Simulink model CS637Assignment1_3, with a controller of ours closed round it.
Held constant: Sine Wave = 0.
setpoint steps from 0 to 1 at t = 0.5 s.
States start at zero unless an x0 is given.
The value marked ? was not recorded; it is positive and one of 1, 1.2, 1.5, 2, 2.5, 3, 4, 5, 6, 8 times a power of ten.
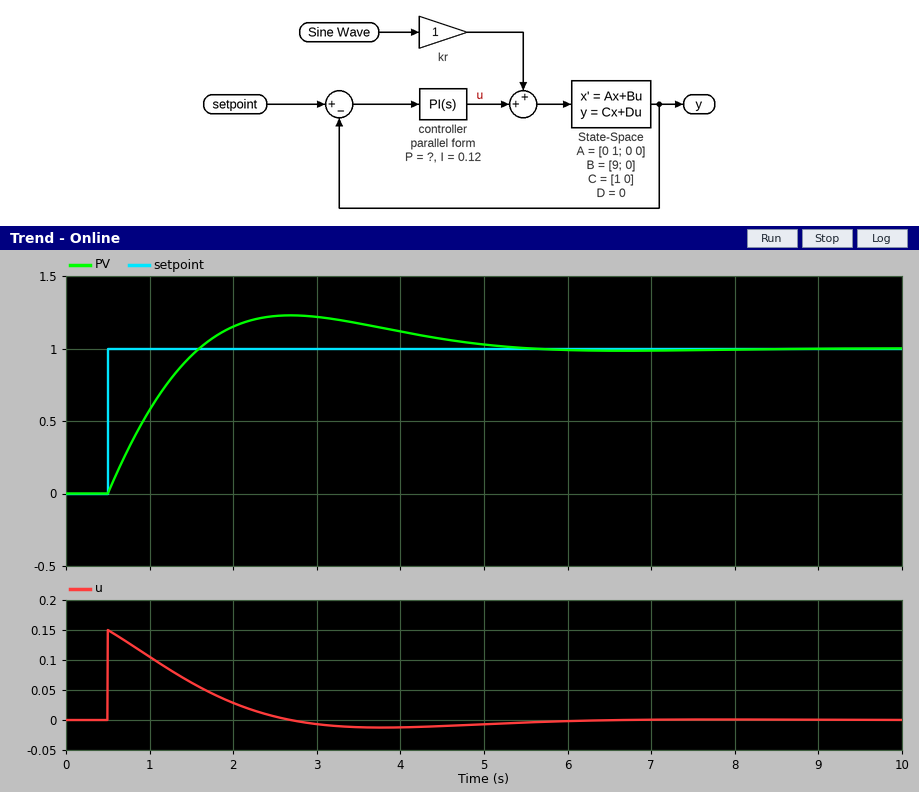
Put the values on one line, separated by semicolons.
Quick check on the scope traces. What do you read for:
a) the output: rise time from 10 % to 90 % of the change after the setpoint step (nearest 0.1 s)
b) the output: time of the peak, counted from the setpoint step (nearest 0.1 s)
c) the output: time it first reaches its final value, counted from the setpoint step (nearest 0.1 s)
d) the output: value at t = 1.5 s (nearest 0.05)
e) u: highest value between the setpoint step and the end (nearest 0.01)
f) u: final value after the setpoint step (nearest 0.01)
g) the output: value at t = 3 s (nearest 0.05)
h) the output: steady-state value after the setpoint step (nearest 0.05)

0.8 s; 2.2 s; 1.1 s; 0.95; 0.15; 0.00; 1.20; 1.00
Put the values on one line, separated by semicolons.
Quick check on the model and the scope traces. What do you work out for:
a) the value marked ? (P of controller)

0.15
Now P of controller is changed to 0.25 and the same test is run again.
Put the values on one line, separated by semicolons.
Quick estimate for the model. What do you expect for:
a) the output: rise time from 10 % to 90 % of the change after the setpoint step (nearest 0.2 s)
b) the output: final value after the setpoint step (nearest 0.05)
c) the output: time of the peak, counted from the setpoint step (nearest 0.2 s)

0.6 s; 1.00; 1.8 s
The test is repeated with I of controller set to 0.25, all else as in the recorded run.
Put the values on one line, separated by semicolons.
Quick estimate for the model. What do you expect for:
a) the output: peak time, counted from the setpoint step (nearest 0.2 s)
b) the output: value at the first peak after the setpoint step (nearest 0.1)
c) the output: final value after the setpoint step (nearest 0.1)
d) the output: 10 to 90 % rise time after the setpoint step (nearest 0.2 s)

1.6 s; 1.3; 1.0; 0.6 s
